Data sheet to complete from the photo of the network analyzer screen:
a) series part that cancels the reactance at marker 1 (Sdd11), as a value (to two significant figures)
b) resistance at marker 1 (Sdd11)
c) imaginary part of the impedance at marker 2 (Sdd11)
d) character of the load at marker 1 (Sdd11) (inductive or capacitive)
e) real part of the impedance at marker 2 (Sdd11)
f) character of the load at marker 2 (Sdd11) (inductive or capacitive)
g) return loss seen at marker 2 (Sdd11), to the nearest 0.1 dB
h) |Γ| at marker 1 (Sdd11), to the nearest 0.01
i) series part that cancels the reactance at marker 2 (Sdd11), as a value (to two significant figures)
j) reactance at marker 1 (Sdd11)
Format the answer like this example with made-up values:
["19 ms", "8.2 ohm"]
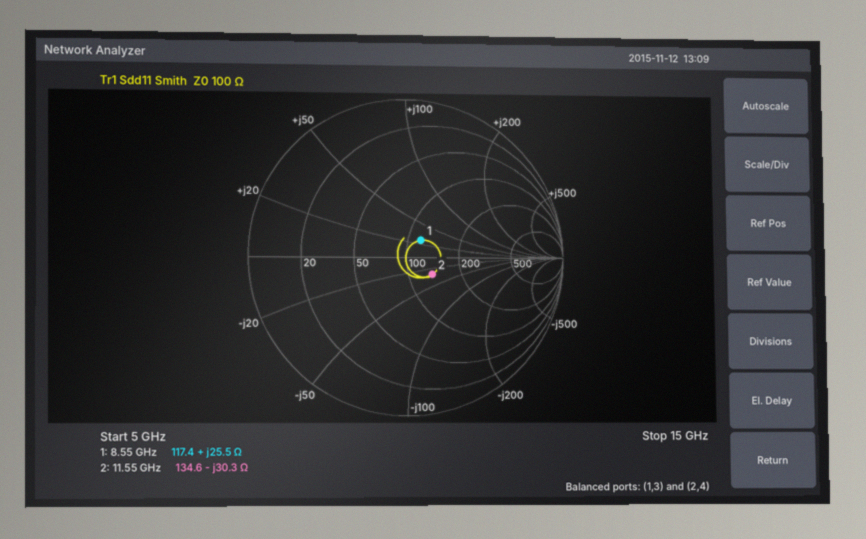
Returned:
["730 fF", "117.4 Ω", "-30.3 Ω", "inductive", "134.6 Ω", "capacitive", "14.2 dB", "0.14", "420 pH", "+25.5 Ω"]
